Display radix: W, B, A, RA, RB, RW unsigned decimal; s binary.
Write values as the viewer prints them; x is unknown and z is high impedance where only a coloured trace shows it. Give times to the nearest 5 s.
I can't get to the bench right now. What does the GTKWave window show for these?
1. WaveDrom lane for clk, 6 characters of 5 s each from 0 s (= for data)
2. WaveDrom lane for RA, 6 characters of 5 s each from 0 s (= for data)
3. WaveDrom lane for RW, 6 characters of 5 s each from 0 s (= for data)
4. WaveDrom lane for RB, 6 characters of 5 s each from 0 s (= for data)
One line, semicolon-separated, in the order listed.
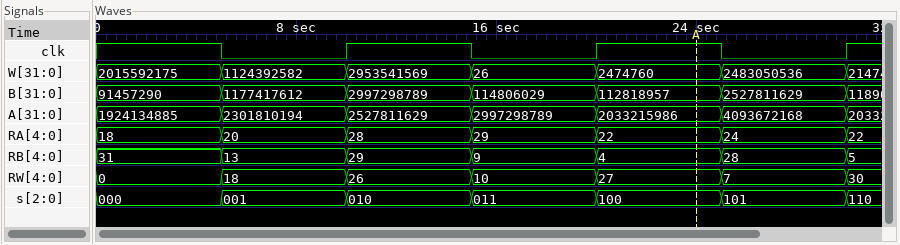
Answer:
{name: 'clk', wave: '101010'}; {name: 'RA', wave: '======', data: '18 20 28 29 22 24'}; {name: 'RW', wave: '======', data: '0 18 26 10 27 7'}; {name: 'RB', wave: '======', data: '31 13 29 9 4 28'}
